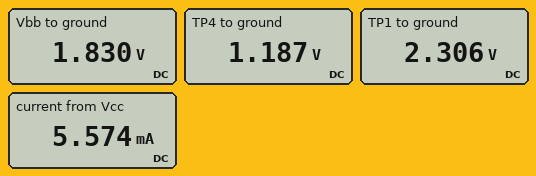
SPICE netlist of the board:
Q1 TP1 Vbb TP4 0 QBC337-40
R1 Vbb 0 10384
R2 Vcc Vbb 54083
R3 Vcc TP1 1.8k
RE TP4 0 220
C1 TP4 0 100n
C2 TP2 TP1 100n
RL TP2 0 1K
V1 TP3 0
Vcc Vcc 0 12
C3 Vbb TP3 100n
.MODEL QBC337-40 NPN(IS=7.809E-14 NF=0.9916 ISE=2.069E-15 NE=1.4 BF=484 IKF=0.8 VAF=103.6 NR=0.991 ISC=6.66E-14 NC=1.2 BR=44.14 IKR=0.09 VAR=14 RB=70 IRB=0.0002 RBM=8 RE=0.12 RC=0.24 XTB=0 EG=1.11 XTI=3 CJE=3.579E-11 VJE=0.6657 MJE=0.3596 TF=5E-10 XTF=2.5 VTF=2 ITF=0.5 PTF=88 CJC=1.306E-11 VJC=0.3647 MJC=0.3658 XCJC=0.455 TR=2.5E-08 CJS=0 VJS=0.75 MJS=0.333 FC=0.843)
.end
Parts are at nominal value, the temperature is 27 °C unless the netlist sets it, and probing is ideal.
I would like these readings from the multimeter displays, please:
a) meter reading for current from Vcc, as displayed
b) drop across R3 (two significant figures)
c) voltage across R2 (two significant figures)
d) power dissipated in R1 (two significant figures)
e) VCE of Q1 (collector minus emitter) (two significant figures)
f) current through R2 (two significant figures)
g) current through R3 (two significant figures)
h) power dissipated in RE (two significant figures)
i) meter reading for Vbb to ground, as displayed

5.574 mA
9.7 V
10 V
320 µW
1.1 V
190 µA
5.4 mA
6.4 mW
1.830 V
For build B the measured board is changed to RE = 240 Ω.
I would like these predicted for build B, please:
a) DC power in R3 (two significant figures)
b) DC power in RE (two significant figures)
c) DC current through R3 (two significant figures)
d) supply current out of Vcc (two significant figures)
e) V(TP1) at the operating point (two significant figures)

45 mW
6.0 mW
5.0 mA
5.2 mA
3.0 V
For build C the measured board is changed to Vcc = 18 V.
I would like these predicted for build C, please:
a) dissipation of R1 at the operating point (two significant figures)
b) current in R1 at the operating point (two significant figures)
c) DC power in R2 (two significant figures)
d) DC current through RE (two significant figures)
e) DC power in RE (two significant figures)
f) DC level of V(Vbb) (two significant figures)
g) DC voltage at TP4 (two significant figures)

660 µW
250 µA
4.4 mW
8.9 mA
17 mW
2.6 V
2.0 V
